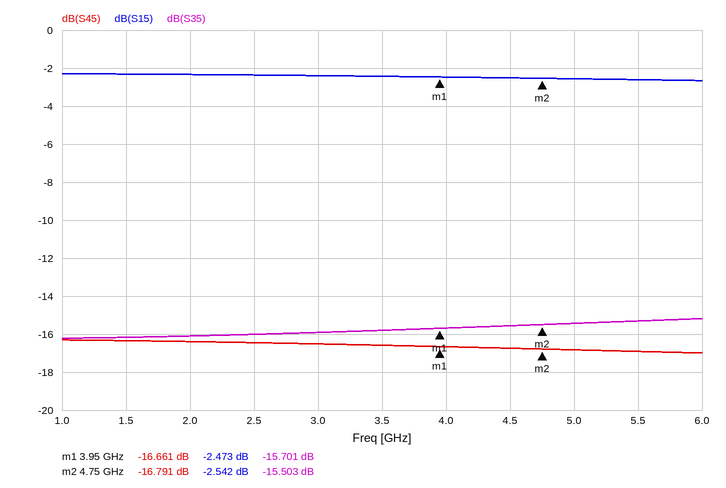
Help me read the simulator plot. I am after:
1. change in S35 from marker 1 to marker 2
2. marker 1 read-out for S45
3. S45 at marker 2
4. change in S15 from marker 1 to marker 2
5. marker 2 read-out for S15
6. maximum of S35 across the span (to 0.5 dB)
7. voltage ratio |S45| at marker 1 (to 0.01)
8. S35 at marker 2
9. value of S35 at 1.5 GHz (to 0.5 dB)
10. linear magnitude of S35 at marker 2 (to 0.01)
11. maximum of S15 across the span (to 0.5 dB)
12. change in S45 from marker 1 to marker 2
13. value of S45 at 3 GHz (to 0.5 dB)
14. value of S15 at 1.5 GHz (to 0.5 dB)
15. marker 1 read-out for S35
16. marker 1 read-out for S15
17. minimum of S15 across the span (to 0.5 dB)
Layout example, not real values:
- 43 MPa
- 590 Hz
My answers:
- 0.198 dB
- -16.661 dB
- -16.791 dB
- -0.069 dB
- -2.542 dB
- -15.0 dB
- 0.15
- -15.503 dB
- -16.0 dB
- 0.17
- -2.5 dB
- -0.130 dB
- -16.5 dB
- -2.5 dB
- -15.701 dB
- -2.473 dB
- -2.5 dB
